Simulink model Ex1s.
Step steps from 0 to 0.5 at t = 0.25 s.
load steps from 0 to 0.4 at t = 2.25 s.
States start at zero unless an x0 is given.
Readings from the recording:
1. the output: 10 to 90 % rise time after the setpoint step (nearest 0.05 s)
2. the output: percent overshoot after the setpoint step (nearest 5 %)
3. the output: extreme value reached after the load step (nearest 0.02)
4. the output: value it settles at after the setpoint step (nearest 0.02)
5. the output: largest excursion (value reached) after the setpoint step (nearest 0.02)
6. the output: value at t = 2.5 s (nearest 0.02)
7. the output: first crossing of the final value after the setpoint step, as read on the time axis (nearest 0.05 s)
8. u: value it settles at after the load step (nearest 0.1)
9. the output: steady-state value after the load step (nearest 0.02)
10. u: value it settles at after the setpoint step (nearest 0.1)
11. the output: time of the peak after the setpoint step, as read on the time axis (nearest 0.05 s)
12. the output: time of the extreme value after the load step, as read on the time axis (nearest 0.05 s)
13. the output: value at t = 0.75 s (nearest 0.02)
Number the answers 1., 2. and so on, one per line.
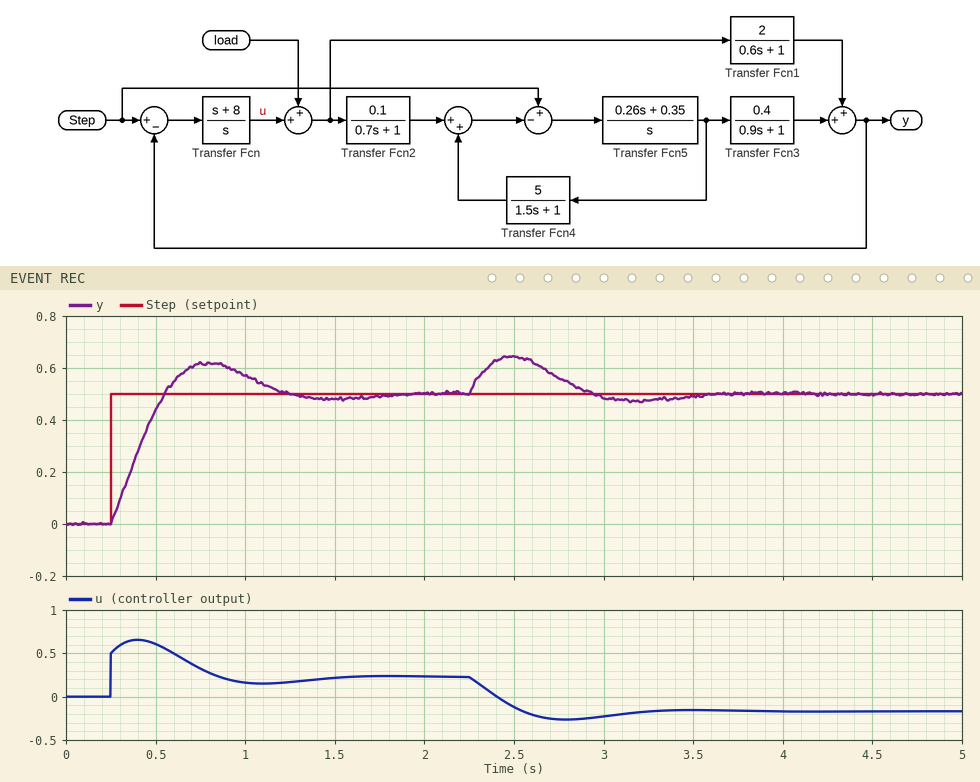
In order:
1. 0.25 s
2. 25 %
3. 0.64
4. 0.50
5. 0.62
6. 0.64
7. 0.55 s
8. -0.2
9. 0.50
10. 0.2
11. 0.80 s
12. 2.50 s
13. 0.62
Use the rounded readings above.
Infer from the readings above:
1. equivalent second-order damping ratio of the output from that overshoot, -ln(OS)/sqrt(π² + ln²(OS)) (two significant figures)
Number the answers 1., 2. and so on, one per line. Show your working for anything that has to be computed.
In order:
1. ln(0.25) = -1.386; 1.386 / sqrt(9.870 + 1.922) = 0.40
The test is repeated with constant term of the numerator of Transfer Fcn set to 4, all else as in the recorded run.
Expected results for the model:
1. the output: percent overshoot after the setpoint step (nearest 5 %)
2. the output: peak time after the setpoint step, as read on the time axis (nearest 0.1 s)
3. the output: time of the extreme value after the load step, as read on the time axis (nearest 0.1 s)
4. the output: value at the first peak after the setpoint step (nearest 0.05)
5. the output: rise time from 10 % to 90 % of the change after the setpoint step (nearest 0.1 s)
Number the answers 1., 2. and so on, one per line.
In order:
1. 10 %
2. 1.0 s
3. 2.6 s
4. 0.55
5. 0.3 s
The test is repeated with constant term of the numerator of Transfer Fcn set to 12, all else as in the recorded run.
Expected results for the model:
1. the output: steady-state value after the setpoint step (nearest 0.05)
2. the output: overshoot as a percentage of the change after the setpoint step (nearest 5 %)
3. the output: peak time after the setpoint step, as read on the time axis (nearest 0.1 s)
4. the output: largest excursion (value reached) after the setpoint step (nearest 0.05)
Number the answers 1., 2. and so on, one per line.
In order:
1. 0.50
2. 30 %
3. 0.7 s
4. 0.65
